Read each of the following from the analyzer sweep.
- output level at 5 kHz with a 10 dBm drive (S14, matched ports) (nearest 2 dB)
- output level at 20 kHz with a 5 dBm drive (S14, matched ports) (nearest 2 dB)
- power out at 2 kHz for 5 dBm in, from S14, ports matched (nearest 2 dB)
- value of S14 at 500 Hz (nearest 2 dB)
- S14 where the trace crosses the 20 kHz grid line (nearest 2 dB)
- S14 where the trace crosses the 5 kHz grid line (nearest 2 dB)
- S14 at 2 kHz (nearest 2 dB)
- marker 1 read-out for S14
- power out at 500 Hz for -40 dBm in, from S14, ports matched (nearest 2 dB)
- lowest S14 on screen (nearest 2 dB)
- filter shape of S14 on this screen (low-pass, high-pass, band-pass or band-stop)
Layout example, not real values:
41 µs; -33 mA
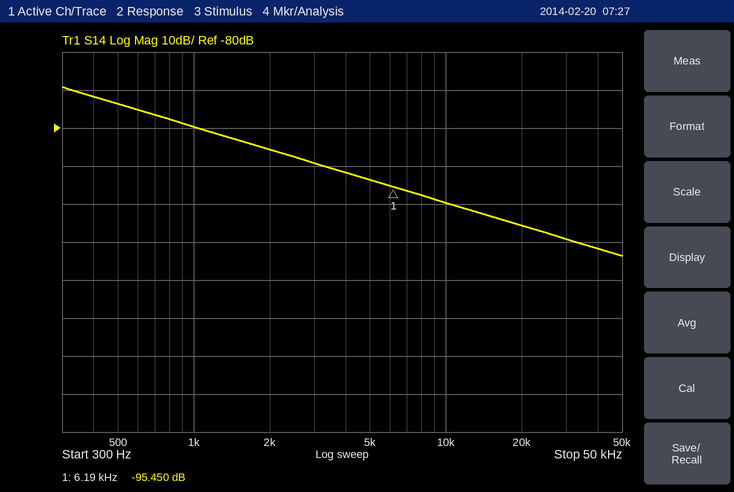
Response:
-84 dBm; -100 dBm; -80 dBm; -74 dB; -106 dB; -94 dB; -86 dB; -95.450 dB; -114 dBm; -114 dB; low-pass
